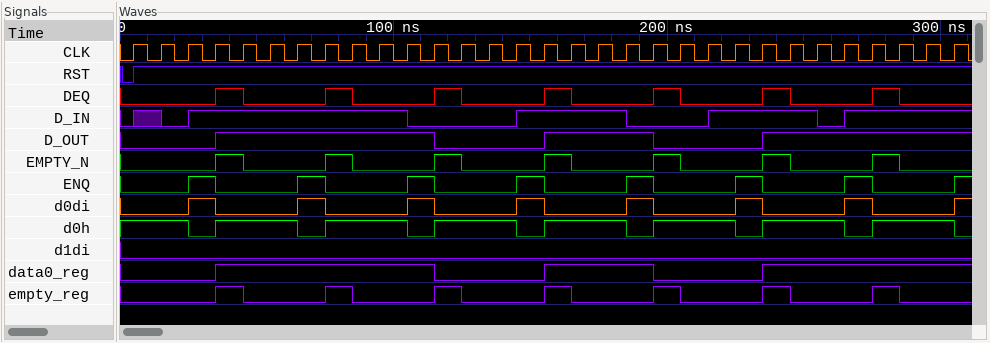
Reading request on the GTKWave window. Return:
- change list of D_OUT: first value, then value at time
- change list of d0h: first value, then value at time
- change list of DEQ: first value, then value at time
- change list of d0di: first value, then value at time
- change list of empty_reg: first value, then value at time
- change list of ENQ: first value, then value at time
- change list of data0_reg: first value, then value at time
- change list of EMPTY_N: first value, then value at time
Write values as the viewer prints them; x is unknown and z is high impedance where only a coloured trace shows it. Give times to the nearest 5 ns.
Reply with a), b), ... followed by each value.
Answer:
a) 0, 1 at 35 ns, 0 at 115 ns, 1 at 155 ns, 0 at 195 ns, 1 at 235 ns
b) 1, 0 at 25 ns, 1 at 35 ns, 0 at 65 ns, 1 at 75 ns, 0 at 105 ns, 1 at 115 ns, 0 at 145 ns, 1 at 155 ns, 0 at 185 ns, 1 at 195 ns, 0 at 225 ns, 1 at 235 ns, 0 at 265 ns, 1 at 275 ns, 0 at 305 ns
c) 0, 1 at 35 ns, 0 at 45 ns, 1 at 75 ns, 0 at 85 ns, 1 at 115 ns, 0 at 125 ns, 1 at 155 ns, 0 at 165 ns, 1 at 195 ns, 0 at 205 ns, 1 at 235 ns, 0 at 245 ns, 1 at 275 ns, 0 at 285 ns
d) 0, 1 at 25 ns, 0 at 35 ns, 1 at 65 ns, 0 at 75 ns, 1 at 105 ns, 0 at 115 ns, 1 at 145 ns, 0 at 155 ns, 1 at 185 ns, 0 at 195 ns, 1 at 225 ns, 0 at 235 ns, 1 at 265 ns, 0 at 275 ns, 1 at 305 ns
e) 0, 1 at 35 ns, 0 at 45 ns, 1 at 75 ns, 0 at 85 ns, 1 at 115 ns, 0 at 125 ns, 1 at 155 ns, 0 at 165 ns, 1 at 195 ns, 0 at 205 ns, 1 at 235 ns, 0 at 245 ns, 1 at 275 ns, 0 at 285 ns
f) 0, 1 at 25 ns, 0 at 35 ns, 1 at 65 ns, 0 at 75 ns, 1 at 105 ns, 0 at 115 ns, 1 at 145 ns, 0 at 155 ns, 1 at 185 ns, 0 at 195 ns, 1 at 225 ns, 0 at 235 ns, 1 at 265 ns, 0 at 275 ns, 1 at 305 ns
g) 0, 1 at 35 ns, 0 at 115 ns, 1 at 155 ns, 0 at 195 ns, 1 at 235 ns
h) 0, 1 at 35 ns, 0 at 45 ns, 1 at 75 ns, 0 at 85 ns, 1 at 115 ns, 0 at 125 ns, 1 at 155 ns, 0 at 165 ns, 1 at 195 ns, 0 at 205 ns, 1 at 235 ns, 0 at 245 ns, 1 at 275 ns, 0 at 285 ns
